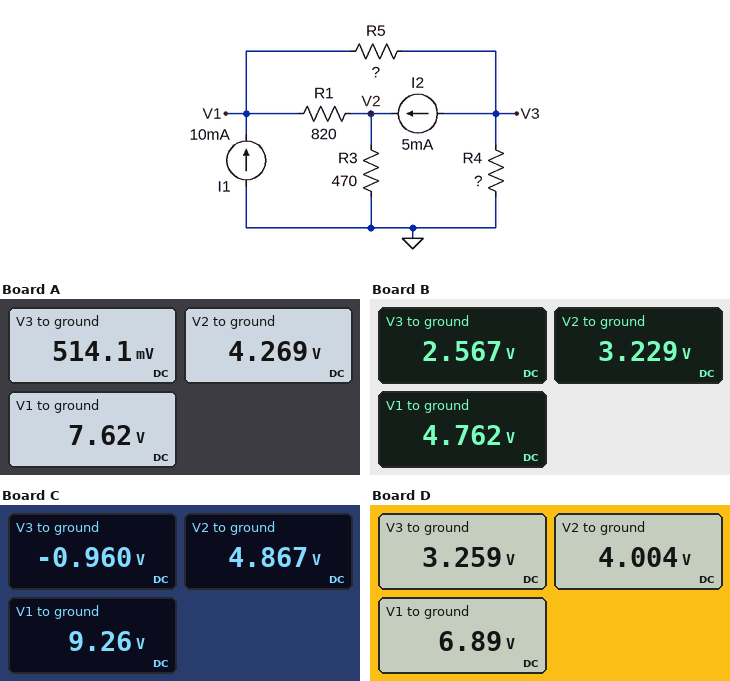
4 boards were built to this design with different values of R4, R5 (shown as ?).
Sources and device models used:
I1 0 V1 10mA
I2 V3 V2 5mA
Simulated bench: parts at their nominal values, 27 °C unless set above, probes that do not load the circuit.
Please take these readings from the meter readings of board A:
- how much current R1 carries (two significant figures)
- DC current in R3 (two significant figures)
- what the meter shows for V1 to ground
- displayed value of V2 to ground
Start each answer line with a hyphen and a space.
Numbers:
- 4.1 mA
- 9.1 mA
- 7.62 V
- 4.269 V
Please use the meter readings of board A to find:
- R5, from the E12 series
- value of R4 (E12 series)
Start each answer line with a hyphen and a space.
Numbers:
- 1.2 kΩ
- 560 Ω
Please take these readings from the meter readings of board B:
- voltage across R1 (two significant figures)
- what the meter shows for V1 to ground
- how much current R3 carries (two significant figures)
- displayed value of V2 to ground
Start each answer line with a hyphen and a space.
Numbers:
- 1.5 V
- 4.762 V
- 6.9 mA
- 3.229 V
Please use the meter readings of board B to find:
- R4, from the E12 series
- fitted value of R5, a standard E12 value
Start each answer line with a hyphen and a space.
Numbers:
- 820 Ω
- 270 Ω
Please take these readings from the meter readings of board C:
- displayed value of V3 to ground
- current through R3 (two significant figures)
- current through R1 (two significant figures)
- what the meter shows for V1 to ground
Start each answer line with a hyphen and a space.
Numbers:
- -0.960 V
- 10 mA
- 5.4 mA
- 9.26 V
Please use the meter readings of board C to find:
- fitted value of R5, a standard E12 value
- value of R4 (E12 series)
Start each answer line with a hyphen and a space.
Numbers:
- 2.2 kΩ
- 2.7 kΩ
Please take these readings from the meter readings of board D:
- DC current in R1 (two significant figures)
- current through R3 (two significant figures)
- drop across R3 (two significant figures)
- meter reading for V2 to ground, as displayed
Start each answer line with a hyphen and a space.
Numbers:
- 3.5 mA
- 8.5 mA
- 4.0 V
- 4.004 V
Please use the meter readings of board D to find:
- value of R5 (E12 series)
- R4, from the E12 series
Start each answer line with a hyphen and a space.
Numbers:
- 560 Ω
- 2.2 kΩ
